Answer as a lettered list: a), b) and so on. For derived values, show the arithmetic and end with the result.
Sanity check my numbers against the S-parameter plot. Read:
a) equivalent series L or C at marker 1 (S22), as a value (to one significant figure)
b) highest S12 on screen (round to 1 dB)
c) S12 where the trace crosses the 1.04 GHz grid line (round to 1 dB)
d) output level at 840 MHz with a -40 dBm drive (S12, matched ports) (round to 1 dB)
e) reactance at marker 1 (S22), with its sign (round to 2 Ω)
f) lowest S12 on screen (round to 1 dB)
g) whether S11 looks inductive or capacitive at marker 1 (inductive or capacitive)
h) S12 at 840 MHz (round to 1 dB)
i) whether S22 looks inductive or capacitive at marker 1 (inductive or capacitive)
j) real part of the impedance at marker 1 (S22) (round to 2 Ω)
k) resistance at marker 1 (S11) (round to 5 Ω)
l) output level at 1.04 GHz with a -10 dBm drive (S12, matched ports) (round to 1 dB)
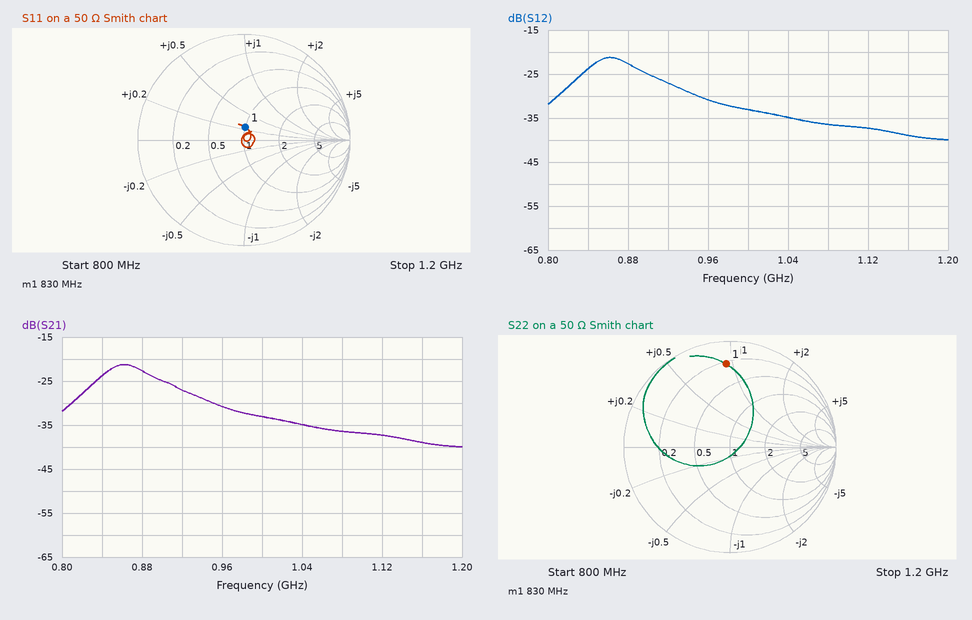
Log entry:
a) L = 46 Ω/(2π × 830 MHz) ≈ 9 nH
b) -21 dB
c) -35 dB
d) -40 dBm + (-24 dB) = -64 dBm
e) +46 Ω
f) -40 dB
g) inductive
h) -24 dB
i) inductive
j) 12 Ω
k) 50 Ω
l) -10 dBm + (-35 dB) = -45 dBm
